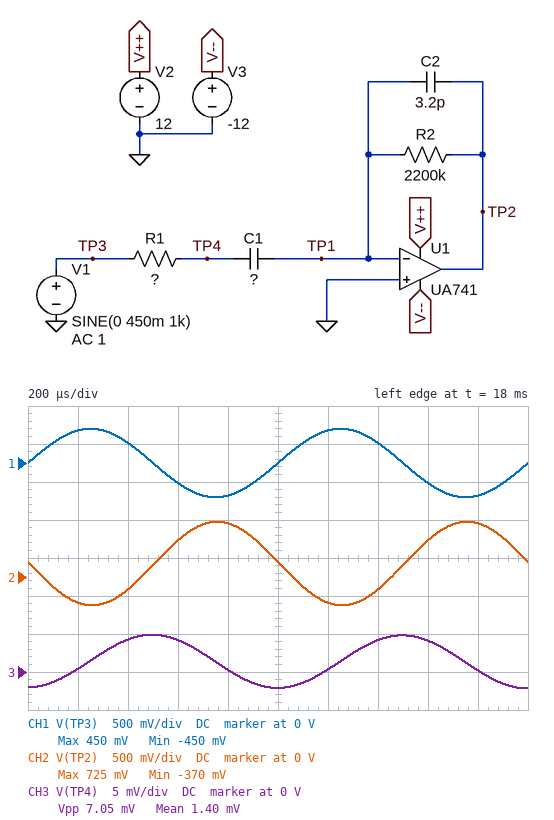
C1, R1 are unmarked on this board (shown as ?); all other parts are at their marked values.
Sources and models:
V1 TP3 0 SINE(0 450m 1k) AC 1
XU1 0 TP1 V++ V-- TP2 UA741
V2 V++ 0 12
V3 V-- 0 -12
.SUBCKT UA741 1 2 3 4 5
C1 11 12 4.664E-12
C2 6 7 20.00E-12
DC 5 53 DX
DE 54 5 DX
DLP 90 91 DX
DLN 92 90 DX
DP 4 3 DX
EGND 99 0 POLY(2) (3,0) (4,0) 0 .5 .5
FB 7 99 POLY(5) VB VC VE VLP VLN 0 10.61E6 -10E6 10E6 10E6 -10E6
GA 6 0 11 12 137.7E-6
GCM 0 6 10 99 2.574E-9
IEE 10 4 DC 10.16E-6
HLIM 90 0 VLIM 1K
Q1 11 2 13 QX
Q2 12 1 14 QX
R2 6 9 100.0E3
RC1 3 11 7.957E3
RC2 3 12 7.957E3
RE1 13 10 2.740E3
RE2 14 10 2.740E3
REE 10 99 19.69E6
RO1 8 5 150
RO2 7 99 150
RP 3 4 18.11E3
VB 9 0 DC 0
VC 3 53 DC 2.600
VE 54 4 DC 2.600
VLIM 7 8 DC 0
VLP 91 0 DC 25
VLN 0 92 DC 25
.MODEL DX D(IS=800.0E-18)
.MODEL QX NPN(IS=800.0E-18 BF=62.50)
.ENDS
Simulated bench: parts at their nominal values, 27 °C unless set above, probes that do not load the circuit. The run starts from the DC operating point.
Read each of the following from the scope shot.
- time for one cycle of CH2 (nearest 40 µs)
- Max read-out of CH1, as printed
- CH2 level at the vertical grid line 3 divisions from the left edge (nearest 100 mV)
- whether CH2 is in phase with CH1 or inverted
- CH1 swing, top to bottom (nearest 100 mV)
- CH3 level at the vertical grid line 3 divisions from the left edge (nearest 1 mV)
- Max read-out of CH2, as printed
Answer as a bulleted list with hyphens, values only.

- 1.00 ms
- 450 mV
- 500 mV
- inverted
- 900 mV
- 4 mV
- 725 mV
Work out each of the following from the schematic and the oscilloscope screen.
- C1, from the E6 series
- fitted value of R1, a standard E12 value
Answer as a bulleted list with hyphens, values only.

- 10 nF
- 1.8 MΩ
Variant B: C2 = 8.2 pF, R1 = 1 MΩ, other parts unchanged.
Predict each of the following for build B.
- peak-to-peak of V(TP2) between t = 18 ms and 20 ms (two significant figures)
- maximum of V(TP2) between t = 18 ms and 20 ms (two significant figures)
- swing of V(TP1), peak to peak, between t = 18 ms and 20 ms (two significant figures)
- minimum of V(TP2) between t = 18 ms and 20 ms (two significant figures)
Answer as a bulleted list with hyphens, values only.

- 2.0 V
- 1.2 V
- 1.8 mV
- -810 mV
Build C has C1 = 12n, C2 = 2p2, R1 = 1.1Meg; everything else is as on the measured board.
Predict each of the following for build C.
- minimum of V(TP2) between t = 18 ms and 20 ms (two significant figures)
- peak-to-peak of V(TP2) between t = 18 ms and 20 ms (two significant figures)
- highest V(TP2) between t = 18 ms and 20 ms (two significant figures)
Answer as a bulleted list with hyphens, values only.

- -720 mV
- 1.8 V
- 1.1 V
